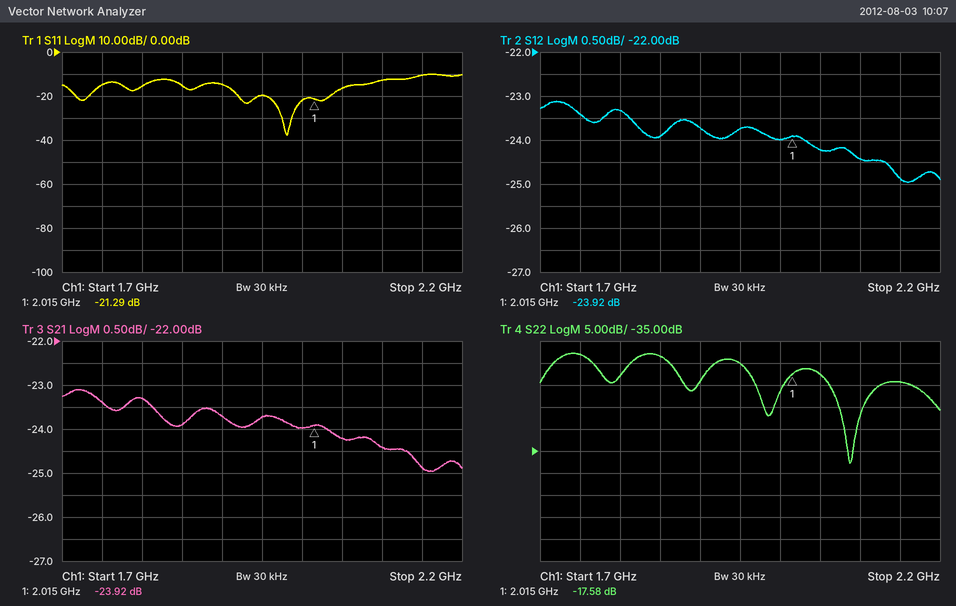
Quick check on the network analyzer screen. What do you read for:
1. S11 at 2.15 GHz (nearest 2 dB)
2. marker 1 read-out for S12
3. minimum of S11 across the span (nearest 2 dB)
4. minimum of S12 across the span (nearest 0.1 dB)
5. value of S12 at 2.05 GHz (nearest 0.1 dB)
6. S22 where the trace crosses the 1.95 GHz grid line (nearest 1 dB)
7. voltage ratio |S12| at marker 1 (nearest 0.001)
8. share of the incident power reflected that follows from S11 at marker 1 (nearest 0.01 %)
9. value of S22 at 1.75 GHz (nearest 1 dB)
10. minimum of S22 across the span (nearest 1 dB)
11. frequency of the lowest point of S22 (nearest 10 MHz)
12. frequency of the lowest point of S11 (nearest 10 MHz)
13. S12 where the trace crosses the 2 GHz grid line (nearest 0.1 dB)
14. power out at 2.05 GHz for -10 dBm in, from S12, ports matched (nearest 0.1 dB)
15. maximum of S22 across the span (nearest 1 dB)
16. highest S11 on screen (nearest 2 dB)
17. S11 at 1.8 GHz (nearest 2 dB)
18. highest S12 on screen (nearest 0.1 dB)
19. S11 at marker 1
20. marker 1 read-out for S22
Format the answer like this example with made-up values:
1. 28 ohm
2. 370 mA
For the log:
1. -10 dB
2. -23.92 dB
3. -38 dB
4. -25.0 dB
5. -24.2 dB
6. -15 dB
7. 0.064
8. 0.74 %
9. -13 dB
10. -38 dB
11. 2.09 GHz
12. 1.98 GHz
13. -24.0 dB
14. -34.2 dBm
15. -13 dB
16. -10 dB
17. -16 dB
18. -23.1 dB
19. -21.29 dB
20. -17.58 dB
